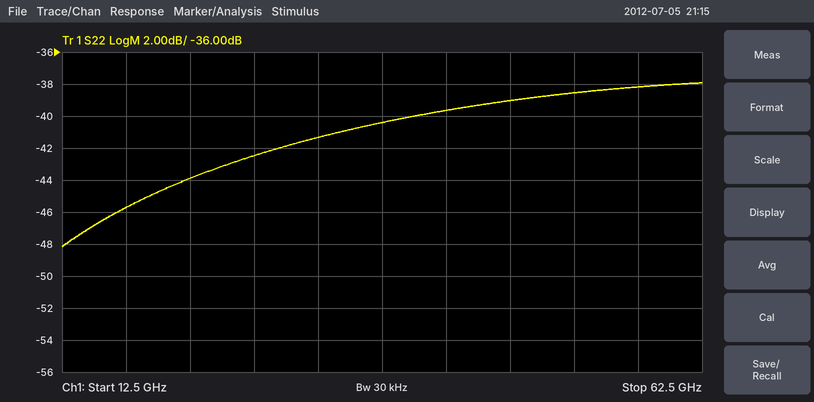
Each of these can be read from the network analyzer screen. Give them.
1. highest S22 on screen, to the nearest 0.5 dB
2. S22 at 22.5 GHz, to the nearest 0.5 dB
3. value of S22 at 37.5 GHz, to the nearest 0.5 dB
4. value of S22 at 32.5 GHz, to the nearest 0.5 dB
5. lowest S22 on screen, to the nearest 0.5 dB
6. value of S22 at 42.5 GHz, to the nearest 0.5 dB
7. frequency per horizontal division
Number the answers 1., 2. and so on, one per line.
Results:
1. -38.0 dB
2. -44.0 dB
3. -40.5 dB
4. -41.5 dB
5. -48.0 dB
6. -39.5 dB
7. 5 GHz
